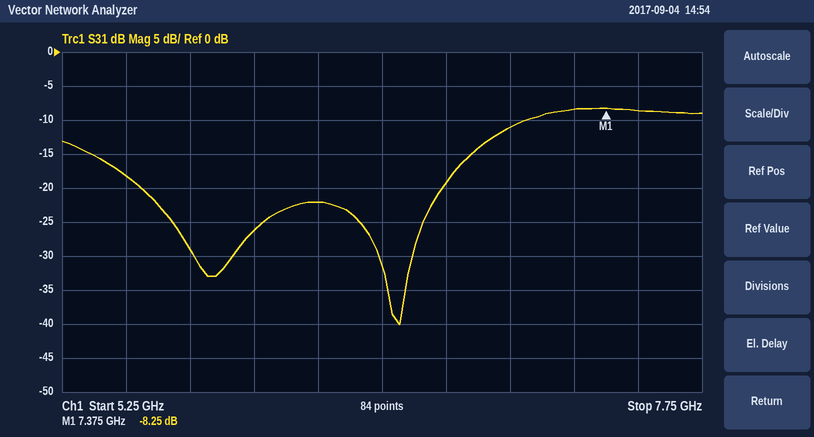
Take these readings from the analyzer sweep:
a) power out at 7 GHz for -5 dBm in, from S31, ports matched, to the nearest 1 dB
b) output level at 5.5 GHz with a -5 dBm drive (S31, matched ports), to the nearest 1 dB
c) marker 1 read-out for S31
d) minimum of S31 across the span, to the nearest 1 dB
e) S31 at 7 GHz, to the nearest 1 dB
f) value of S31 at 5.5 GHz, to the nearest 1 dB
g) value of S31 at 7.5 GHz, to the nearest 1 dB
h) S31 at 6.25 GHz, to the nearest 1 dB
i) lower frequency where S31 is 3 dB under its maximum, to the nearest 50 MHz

-16 dBm
-23 dBm
-8.25 dB
-40 dB
-11 dB
-18 dB
-9 dB
-22 dB
7.00 GHz
